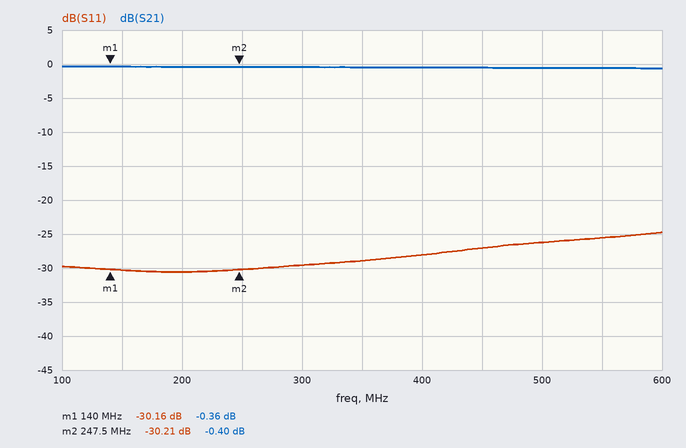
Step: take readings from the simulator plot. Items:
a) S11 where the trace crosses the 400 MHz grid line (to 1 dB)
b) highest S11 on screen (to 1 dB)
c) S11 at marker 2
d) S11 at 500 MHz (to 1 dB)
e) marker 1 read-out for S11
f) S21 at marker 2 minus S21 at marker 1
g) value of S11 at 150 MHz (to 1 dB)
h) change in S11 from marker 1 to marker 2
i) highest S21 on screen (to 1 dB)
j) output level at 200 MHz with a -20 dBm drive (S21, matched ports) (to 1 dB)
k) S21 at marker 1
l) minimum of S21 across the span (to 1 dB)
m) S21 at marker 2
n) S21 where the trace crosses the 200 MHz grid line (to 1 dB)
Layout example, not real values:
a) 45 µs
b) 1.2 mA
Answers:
a) -28 dB
b) -25 dB
c) -30.21 dB
d) -26 dB
e) -30.16 dB
f) -0.04 dB
g) -30 dB
h) -0.05 dB
i) 0 dB
j) -20 dBm
k) -0.36 dB
l) -1 dB
m) -0.40 dB
n) 0 dB
